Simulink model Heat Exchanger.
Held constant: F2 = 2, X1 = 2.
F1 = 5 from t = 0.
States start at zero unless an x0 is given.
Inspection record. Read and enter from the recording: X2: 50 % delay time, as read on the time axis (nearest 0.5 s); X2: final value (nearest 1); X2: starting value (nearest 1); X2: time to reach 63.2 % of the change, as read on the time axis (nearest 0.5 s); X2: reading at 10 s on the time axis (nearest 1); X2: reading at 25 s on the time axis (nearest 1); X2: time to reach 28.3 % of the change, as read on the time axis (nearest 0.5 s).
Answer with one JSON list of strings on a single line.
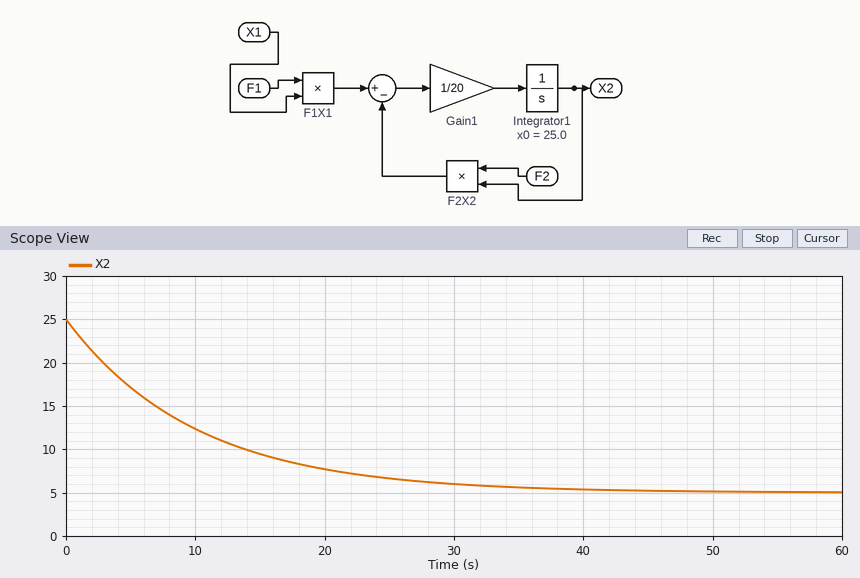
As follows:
["7.0 s", "5", "25", "10.0 s", "12", "7", "3.5 s"]
